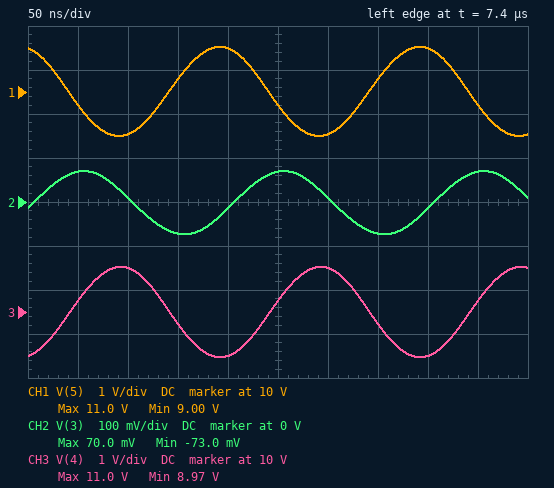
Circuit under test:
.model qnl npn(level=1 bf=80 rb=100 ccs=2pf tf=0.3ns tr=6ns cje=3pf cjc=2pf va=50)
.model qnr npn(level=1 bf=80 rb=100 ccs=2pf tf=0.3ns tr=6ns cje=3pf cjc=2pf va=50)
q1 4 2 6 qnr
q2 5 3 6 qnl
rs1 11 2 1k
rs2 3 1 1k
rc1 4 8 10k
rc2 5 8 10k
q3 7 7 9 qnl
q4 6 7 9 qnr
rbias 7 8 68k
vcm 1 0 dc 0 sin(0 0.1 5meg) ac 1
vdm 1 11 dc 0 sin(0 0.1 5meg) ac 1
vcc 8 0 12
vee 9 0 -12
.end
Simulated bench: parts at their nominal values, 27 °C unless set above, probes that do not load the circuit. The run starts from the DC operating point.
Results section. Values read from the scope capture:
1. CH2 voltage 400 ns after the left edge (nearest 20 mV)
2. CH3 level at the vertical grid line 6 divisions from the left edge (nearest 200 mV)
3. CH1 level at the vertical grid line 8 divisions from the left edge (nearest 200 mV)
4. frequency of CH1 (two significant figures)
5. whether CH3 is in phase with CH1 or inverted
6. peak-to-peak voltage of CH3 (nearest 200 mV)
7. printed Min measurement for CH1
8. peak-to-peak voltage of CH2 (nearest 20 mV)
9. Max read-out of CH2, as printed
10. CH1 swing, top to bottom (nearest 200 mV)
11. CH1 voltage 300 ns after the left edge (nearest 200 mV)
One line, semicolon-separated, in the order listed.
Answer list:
-20 mV; 11.0 V; 11.0 V; 5.0 MHz; inverted; 2.0 V; 9.00 V; 140 mV; 70.0 mV; 2.0 V; 9.0 V
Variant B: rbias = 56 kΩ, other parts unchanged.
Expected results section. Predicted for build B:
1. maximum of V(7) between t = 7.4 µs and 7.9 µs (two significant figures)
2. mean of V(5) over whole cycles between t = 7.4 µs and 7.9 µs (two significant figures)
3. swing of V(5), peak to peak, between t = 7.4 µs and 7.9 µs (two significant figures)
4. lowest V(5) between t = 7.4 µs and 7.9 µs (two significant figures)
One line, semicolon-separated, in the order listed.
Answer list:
-11 V; 9.6 V; 2.2 V; 8.5 V
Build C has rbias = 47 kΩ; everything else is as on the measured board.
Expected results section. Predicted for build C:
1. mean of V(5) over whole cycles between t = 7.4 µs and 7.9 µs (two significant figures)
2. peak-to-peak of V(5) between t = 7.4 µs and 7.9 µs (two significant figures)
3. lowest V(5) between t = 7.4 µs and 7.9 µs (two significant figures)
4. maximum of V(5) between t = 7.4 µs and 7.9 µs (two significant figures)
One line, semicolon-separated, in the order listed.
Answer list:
9.1 V; 2.3 V; 8.0 V; 10 V
